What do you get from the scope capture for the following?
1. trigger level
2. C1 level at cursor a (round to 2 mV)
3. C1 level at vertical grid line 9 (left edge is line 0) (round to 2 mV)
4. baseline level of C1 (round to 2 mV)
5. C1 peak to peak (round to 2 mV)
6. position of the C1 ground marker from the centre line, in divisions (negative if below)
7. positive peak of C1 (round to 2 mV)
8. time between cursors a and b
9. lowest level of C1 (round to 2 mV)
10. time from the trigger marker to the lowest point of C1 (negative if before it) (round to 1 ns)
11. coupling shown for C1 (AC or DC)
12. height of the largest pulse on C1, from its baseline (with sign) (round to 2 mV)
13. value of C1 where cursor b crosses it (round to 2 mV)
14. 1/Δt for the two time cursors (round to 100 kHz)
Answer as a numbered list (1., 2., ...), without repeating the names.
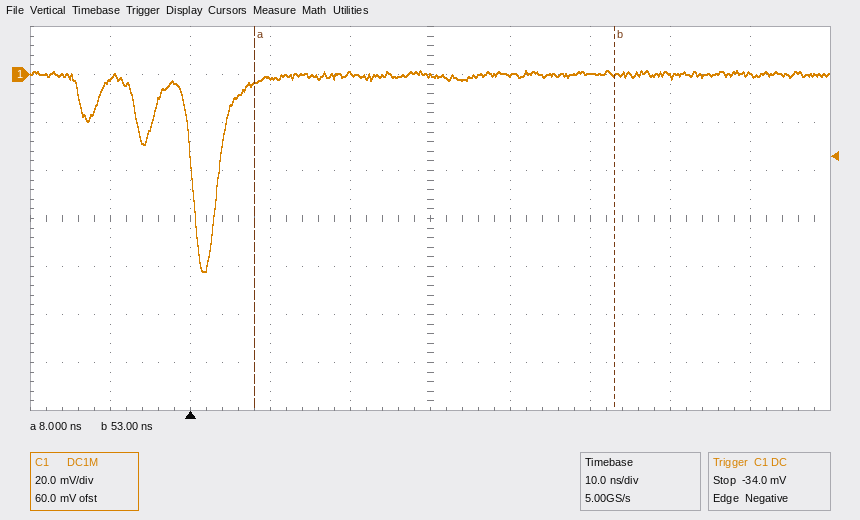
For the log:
1. -34.0 mV
2. -4 mV
3. 0 mV
4. 0 mV
5. 84 mV
6. +3.0 div
7. 2 mV
8. 45 ns
9. -82 mV
10. +2 ns
11. DC
12. -82 mV
13. 0 mV
14. 22.2 MHz
